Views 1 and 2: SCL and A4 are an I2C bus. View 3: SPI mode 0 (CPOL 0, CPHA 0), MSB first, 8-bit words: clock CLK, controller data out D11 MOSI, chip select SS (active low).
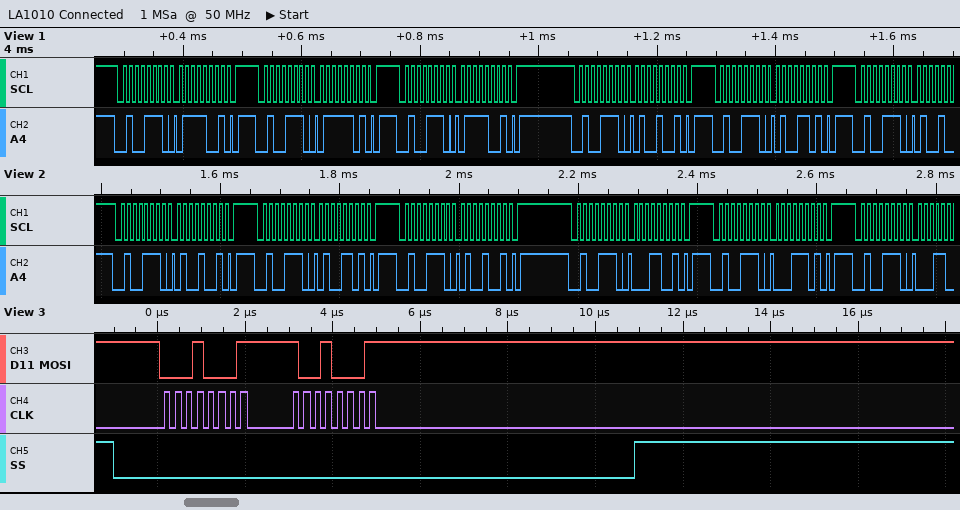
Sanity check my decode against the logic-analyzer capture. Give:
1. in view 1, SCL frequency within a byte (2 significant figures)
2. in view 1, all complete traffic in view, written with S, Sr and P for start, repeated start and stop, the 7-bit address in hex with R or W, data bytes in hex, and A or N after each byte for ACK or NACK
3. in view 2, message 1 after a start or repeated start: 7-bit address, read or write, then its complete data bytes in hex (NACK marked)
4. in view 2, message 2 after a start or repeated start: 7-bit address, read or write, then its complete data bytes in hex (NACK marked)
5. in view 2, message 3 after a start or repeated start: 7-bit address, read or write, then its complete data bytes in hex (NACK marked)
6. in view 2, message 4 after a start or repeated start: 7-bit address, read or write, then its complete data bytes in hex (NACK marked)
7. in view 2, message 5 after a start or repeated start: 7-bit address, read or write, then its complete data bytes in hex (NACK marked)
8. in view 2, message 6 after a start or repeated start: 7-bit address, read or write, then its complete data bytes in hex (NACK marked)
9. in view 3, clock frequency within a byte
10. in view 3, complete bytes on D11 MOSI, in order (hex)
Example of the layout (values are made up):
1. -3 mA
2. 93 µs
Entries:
1. 100 kHz
2. S 27W A 79 A P S 27W A 7D A P S 27W A 79 A P S 27W A 49 A P S 27W A 4D A P S 27W A
3. 0x27 write: 49
4. 0x27 write: 4D
5. 0x27 write: 49
6. 0x27 write: 19
7. 0x27 write: 1D
8. 0x27 write
9. 4 MHz
10. 11 91
